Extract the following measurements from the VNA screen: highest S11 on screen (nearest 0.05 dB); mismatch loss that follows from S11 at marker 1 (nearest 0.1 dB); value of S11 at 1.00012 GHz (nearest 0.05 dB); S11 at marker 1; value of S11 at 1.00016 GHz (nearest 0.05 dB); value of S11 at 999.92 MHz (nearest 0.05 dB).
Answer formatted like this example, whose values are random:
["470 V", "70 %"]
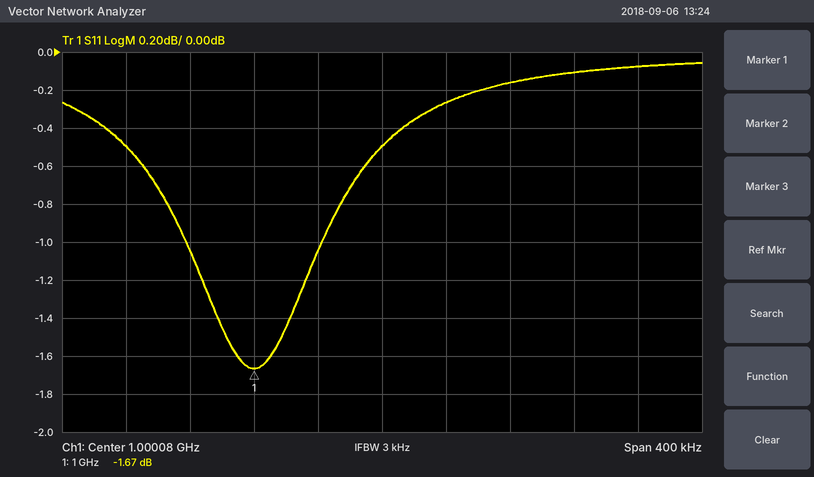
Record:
["-0.05 dB", "5.0 dB", "-0.25 dB", "-1.67 dB", "-0.15 dB", "-0.50 dB"]
